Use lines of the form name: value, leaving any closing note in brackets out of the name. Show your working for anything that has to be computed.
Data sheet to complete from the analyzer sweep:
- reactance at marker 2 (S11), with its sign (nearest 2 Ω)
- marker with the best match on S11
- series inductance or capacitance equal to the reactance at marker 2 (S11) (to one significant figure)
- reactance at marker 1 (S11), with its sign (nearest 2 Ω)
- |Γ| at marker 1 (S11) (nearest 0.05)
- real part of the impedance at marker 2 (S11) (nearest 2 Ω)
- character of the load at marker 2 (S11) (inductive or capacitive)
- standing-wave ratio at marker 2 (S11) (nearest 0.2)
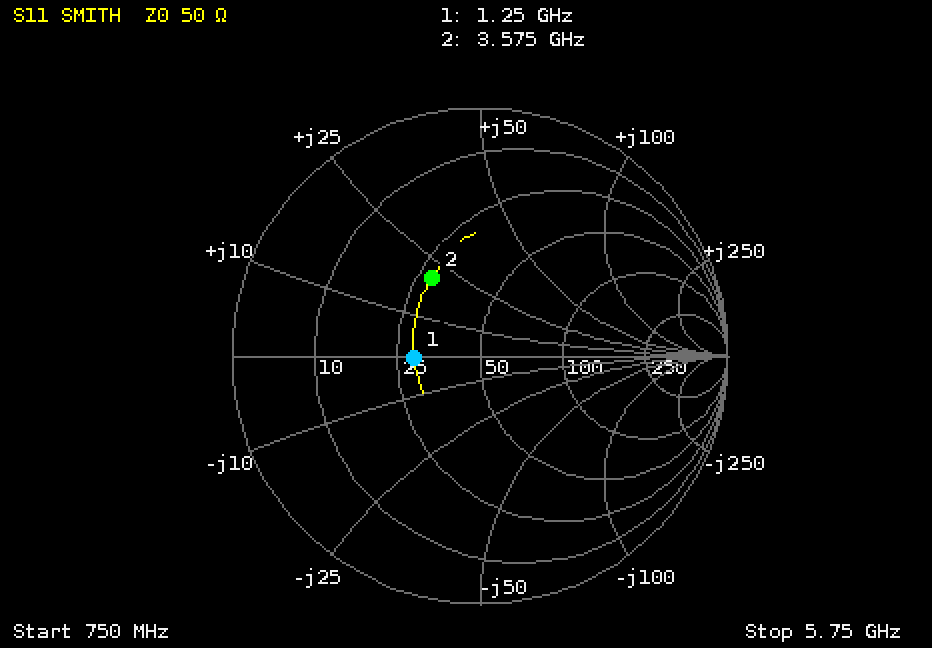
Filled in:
reactance at marker 2 (S11), with its sign: +20 Ω
marker with the best match on S11: marker 1
series inductance or capacitance equal to the reactance at marker 2 (S11): L = 20 Ω/(2π × 3.575 GHz) ≈ 890 pH, so 900 pH to one significant figure
reactance at marker 1 (S11), with its sign: 0 Ω
|Γ| at marker 1 (S11): 0.25
real part of the impedance at marker 2 (S11): 28 Ω
character of the load at marker 2 (S11): inductive
standing-wave ratio at marker 2 (S11): 2.2
